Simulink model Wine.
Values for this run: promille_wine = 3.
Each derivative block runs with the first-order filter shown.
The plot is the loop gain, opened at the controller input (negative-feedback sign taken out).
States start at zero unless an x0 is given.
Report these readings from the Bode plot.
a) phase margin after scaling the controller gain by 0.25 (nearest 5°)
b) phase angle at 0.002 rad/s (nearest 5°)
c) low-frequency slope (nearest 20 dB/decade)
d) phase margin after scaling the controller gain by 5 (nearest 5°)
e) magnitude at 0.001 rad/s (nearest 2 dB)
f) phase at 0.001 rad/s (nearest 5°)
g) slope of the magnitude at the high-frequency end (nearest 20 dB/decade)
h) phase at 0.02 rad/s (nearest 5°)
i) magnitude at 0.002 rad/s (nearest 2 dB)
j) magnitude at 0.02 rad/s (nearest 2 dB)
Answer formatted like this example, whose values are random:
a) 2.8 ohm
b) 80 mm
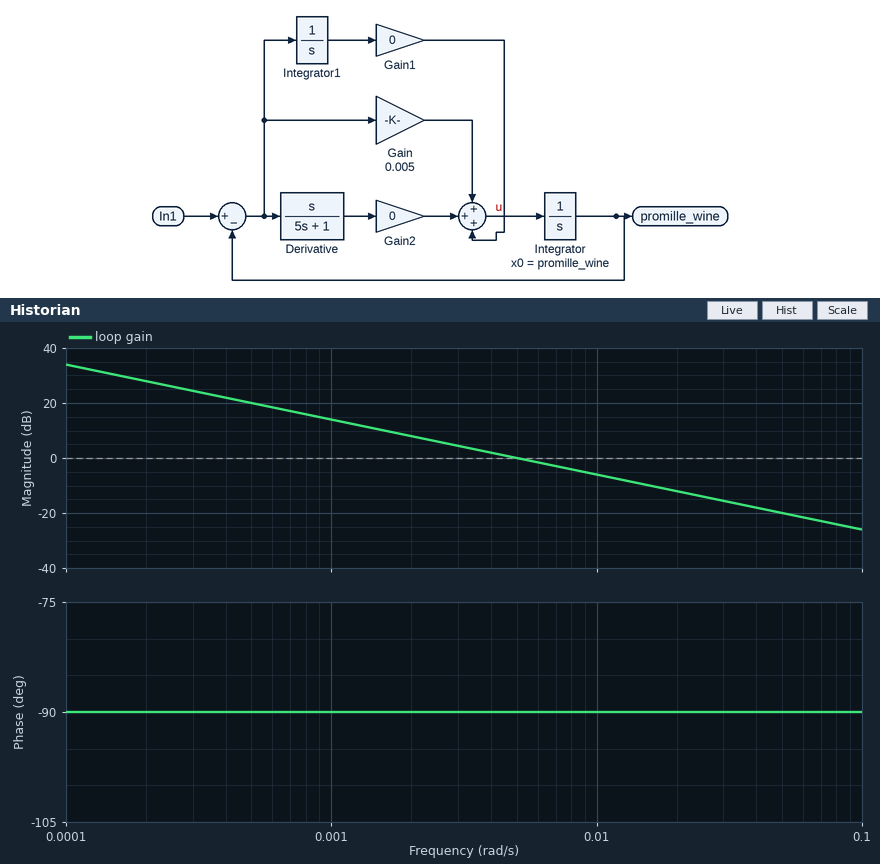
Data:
a) 90°
b) -90°
c) -20 dB/decade
d) 90°
e) 14 dB
f) -90°
g) -20 dB/decade
h) -90°
i) 8 dB
j) -12 dB
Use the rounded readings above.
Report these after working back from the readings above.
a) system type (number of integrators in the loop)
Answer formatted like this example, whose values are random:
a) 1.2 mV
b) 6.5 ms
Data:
a) 1
